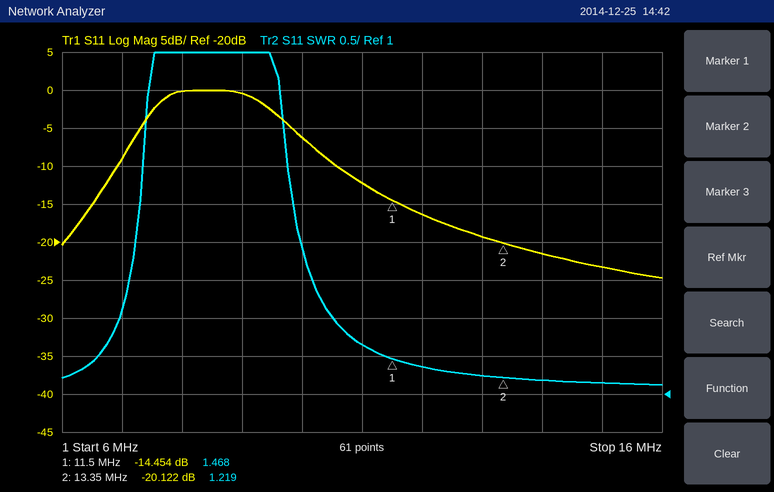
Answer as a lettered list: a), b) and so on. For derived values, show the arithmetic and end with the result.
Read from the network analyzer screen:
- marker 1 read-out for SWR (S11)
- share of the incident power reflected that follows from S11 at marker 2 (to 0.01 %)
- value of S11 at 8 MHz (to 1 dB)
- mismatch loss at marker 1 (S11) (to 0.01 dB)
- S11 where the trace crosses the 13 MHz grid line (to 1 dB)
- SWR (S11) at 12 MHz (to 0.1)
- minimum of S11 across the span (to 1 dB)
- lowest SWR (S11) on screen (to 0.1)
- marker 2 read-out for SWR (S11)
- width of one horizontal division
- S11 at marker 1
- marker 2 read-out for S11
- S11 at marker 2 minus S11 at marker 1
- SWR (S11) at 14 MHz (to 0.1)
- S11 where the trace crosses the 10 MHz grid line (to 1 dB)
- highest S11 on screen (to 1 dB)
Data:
a) 1.468
b) 10^(-20.122/10) ≈ 0.97 %
c) 0 dB
d) −10 log10(1 − 10^(-14.454/10)) ≈ 0.16 dB
e) -19 dB
f) 1.4
g) -25 dB
h) 1.1
i) 1.219
j) 1 MHz
k) -14.454 dB
l) -20.122 dB
m) -20.122 − (-14.454) = -5.668 dB
n) 1.2
o) -6 dB
p) 0 dB
